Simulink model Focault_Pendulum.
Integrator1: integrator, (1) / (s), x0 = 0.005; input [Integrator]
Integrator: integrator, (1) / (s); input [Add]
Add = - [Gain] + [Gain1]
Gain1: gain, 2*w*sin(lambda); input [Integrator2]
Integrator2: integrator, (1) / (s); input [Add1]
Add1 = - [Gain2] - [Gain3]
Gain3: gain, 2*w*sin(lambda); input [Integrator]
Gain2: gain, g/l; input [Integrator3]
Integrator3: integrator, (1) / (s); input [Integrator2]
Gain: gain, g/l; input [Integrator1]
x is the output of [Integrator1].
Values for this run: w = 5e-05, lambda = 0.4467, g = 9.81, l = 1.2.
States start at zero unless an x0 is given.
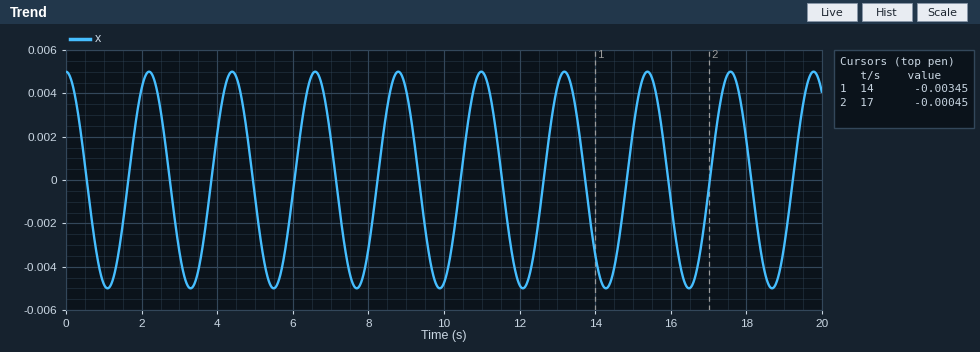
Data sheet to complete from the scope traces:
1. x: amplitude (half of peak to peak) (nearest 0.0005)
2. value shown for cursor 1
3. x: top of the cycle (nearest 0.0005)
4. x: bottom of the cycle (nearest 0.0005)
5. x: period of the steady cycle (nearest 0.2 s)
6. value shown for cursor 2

0.0050
-0.00345
0.0050
-0.0050
2.2 s
-0.00045
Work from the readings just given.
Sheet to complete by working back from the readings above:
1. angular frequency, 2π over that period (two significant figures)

2.9 rad/s
